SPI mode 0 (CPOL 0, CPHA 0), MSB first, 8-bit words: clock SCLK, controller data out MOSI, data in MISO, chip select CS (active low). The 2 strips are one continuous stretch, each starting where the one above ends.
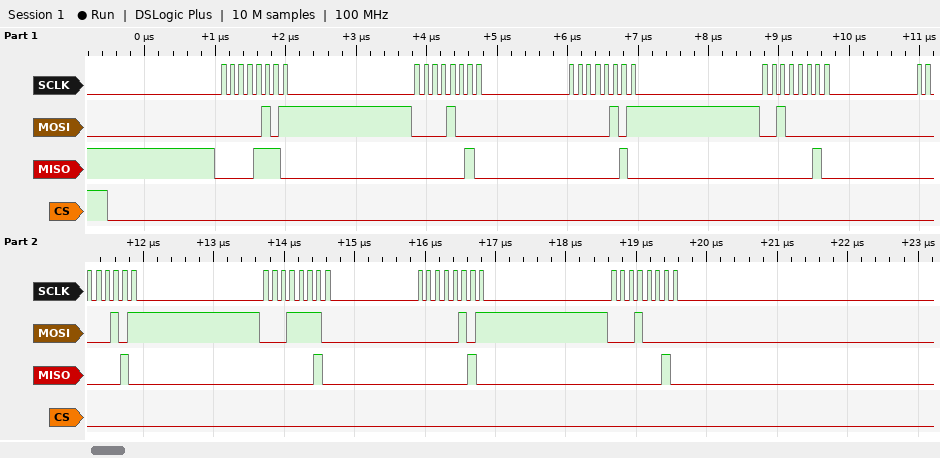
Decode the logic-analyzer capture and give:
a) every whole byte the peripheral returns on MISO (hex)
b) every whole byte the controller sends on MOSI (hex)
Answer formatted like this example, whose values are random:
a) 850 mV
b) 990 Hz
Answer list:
a) 0x0E 0x02 0x02 0x02 0x02 0x02 0x02 0x02
b) 0x05 0x08 0x05 0x20 0x05 0x1E 0x05 0x10
